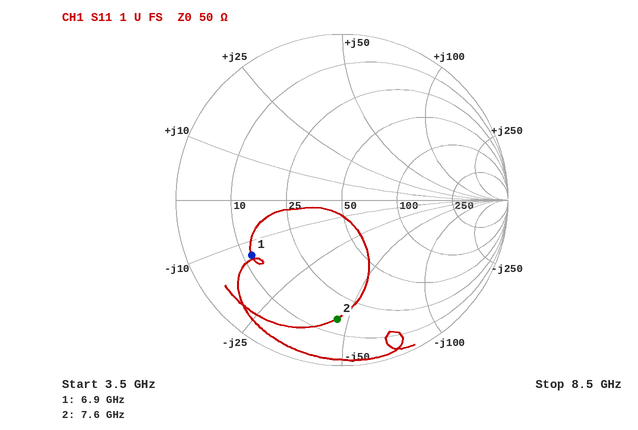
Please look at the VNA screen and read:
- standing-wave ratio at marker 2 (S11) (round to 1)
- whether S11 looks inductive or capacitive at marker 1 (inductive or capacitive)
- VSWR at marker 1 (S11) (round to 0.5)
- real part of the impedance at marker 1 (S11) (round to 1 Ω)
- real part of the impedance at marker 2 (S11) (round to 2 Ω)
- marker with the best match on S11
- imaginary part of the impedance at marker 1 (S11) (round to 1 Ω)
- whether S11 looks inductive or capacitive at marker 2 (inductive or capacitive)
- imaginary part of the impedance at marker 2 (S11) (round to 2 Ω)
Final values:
6
capacitive
4.5
12 Ω
16 Ω
marker 1
-13 Ω
capacitive
-46 Ω
